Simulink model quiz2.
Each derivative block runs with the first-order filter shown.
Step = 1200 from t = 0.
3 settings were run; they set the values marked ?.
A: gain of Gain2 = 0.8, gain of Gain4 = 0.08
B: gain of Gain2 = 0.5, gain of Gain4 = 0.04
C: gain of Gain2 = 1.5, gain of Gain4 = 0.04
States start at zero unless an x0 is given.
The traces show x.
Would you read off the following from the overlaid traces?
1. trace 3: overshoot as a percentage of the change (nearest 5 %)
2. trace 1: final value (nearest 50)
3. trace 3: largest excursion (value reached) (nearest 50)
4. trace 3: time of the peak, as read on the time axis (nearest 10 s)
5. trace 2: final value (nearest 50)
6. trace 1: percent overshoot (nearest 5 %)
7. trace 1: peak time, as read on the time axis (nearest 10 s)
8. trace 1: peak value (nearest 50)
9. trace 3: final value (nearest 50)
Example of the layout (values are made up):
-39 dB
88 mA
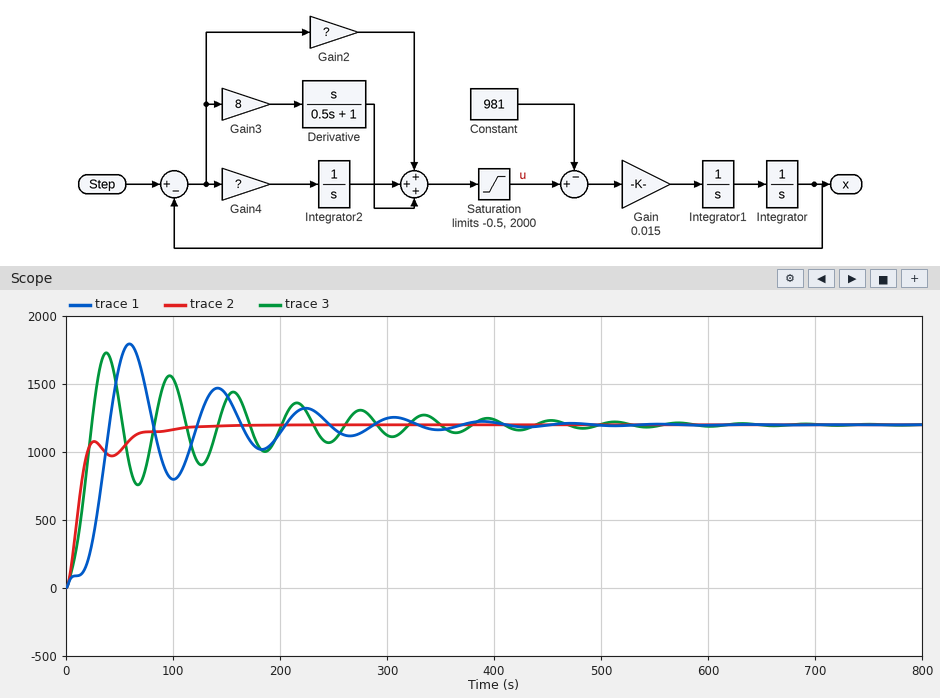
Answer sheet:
45 %
1200
1750
40 s
1200
50 %
60 s
1800
1200
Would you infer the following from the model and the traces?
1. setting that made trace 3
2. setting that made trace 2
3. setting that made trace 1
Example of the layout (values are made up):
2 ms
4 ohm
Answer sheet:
A
C
B
